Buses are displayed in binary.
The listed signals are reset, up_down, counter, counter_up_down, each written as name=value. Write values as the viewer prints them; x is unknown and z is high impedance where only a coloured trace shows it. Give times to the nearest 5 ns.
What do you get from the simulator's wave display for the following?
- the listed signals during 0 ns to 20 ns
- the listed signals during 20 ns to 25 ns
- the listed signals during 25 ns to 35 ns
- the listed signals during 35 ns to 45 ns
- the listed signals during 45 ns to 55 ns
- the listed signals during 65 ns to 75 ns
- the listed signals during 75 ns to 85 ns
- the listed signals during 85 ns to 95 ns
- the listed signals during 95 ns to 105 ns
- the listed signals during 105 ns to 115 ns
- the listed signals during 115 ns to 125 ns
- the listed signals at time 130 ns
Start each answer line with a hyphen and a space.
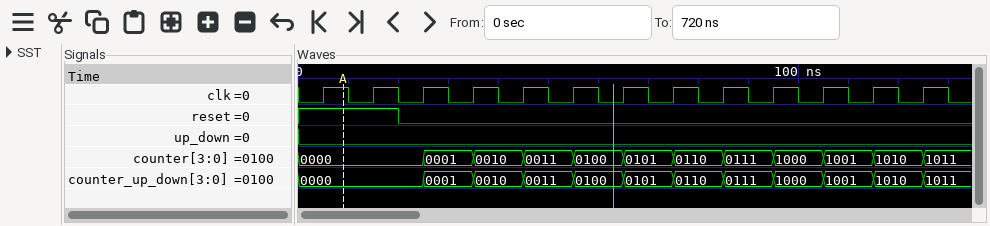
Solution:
- reset=1, up_down=0, counter=0000, counter_up_down=0000
- reset=0, up_down=0, counter=0000, counter_up_down=0000
- reset=0, up_down=0, counter=0001, counter_up_down=0001
- reset=0, up_down=0, counter=0010, counter_up_down=0010
- reset=0, up_down=0, counter=0011, counter_up_down=0011
- reset=0, up_down=0, counter=0101, counter_up_down=0101
- reset=0, up_down=0, counter=0110, counter_up_down=0110
- reset=0, up_down=0, counter=0111, counter_up_down=0111
- reset=0, up_down=0, counter=1000, counter_up_down=1000
- reset=0, up_down=0, counter=1001, counter_up_down=1001
- reset=0, up_down=0, counter=1010, counter_up_down=1010
- reset=0, up_down=0, counter=1011, counter_up_down=1011
